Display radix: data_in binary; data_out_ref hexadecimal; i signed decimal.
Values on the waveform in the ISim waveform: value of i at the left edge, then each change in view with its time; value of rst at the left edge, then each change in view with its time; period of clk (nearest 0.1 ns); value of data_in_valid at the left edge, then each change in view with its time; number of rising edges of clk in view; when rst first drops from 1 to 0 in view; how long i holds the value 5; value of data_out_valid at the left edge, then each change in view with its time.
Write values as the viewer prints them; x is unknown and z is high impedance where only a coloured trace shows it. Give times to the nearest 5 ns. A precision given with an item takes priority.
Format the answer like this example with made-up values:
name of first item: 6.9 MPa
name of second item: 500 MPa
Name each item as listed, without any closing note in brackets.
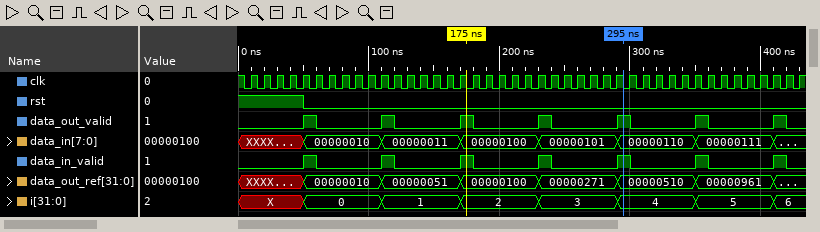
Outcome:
value of i at the left edge, then each change in view with its time: X, 0 at 50 ns, 1 at 110 ns, 2 at 170 ns, 3 at 230 ns, 4 at 290 ns, 5 at 350 ns, 6 at 410 ns
value of rst at the left edge, then each change in view with its time: 1, 0 at 50 ns
period of clk: 10 ns
value of data_in_valid at the left edge, then each change in view with its time: 0, 1 at 50 ns, 0 at 60 ns, 1 at 110 ns, 0 at 120 ns, 1 at 170 ns, 0 at 180 ns, 1 at 230 ns, 0 at 240 ns, 1 at 290 ns, 0 at 300 ns, 1 at 350 ns, 0 at 360 ns, 1 at 410 ns, 0 at 420 ns
number of rising edges of clk in view: 43
when rst first drops from 1 to 0 in view: 50 ns
how long i holds the value 5: 60 ns
value of data_out_valid at the left edge, then each change in view with its time: 0, 1 at 50 ns, 0 at 60 ns, 1 at 110 ns, 0 at 120 ns, 1 at 170 ns, 0 at 180 ns, 1 at 230 ns, 0 at 240 ns, 1 at 290 ns, 0 at 300 ns, 1 at 350 ns, 0 at 360 ns, 1 at 410 ns, 0 at 420 ns
